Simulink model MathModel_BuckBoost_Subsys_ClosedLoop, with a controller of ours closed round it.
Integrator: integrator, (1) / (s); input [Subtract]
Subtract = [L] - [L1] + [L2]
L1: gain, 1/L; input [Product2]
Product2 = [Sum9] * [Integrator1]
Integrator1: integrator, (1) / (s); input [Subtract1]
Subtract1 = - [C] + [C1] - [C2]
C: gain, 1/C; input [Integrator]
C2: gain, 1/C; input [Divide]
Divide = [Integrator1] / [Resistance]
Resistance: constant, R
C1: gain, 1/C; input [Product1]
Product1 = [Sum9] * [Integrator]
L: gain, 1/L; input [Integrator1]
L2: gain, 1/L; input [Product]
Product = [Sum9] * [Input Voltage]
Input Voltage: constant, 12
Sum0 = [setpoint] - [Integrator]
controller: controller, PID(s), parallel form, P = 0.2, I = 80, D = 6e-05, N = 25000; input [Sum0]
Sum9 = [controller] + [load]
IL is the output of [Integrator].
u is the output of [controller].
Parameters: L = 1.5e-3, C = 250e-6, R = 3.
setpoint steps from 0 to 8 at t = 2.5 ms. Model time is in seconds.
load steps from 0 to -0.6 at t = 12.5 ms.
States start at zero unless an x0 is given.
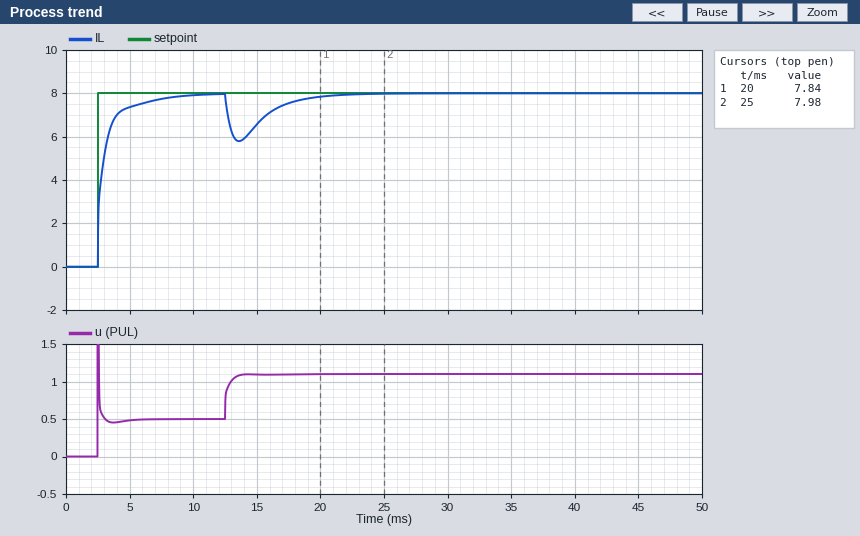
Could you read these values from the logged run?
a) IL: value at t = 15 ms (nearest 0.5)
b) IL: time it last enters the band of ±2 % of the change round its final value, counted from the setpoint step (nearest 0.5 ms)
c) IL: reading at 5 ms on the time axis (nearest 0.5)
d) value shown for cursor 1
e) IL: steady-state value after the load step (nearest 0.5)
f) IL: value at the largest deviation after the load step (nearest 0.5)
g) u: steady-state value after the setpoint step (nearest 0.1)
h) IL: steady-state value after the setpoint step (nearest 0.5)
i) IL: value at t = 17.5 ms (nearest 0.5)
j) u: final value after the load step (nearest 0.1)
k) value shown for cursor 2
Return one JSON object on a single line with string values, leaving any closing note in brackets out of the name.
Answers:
{"IL: value at t = 15 ms": "6.5", "IL: time it last enters the band of ±2 % of the change round its final value, counted from the setpoint step": "6.0 ms", "IL: reading at 5 ms on the time axis": "7.5", "value shown for cursor 1": "7.84", "IL: steady-state value after the load step": "8.0", "IL: value at the largest deviation after the load step": "6.0", "u: steady-state value after the setpoint step": "0.5", "IL: steady-state value after the setpoint step": "8.0", "IL: value at t = 17.5 ms": "7.5", "u: final value after the load step": "1.1", "value shown for cursor 2": "7.98"}
